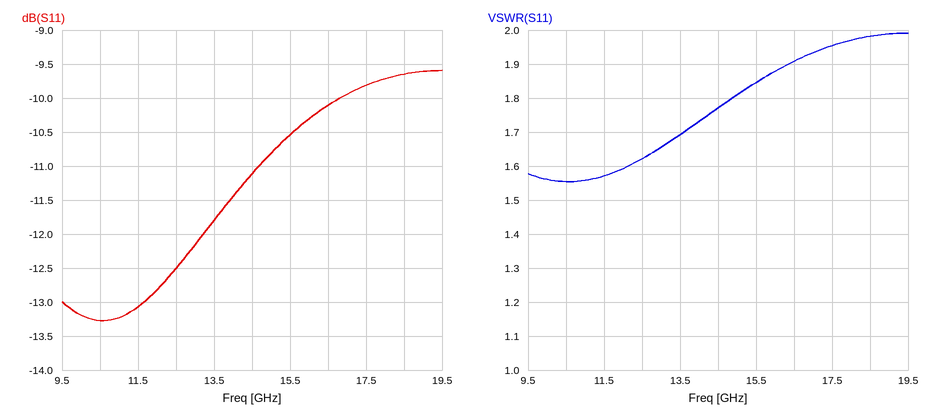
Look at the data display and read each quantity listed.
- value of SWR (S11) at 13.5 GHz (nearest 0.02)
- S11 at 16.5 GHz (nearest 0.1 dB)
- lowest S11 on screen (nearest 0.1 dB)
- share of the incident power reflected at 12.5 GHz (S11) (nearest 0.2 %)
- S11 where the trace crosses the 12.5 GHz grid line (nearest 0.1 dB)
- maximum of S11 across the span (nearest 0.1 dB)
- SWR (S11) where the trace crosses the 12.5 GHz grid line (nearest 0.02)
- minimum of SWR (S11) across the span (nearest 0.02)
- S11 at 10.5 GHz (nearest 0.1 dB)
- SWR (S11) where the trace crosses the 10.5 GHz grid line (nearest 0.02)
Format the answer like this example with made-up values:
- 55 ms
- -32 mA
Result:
- 1.70
- -10.1 dB
- -13.3 dB
- 5.6 %
- -12.5 dB
- -9.6 dB
- 1.62
- 1.56
- -13.3 dB
- 1.56
